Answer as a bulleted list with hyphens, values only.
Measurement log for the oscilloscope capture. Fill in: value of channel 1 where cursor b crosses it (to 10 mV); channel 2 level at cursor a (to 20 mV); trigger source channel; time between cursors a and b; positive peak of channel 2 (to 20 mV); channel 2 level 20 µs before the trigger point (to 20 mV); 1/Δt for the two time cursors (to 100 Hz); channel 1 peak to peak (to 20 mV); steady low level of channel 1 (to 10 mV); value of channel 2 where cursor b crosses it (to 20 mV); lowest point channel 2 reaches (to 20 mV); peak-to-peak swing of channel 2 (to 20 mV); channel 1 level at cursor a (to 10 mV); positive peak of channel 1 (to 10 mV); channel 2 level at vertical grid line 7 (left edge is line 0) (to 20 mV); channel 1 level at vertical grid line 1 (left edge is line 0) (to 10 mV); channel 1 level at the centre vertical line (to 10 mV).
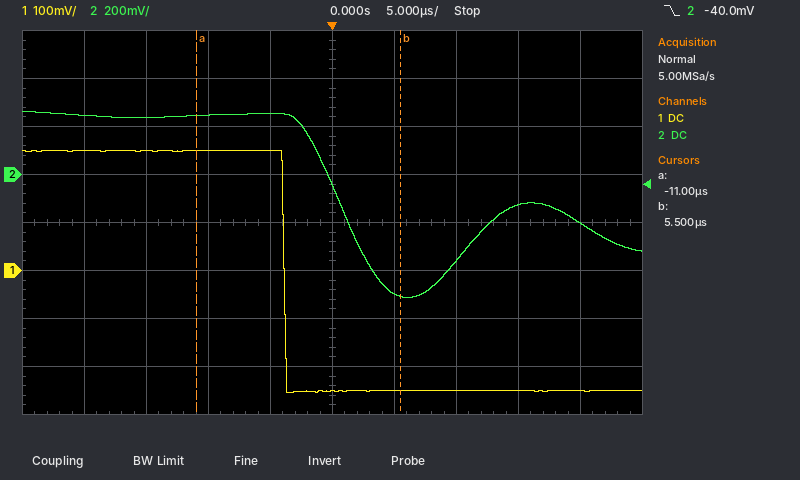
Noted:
- -250 mV
- 240 mV
- channel 2
- 16.5 µs
- 260 mV
- 240 mV
- 60.6 kHz
- 500 mV
- -250 mV
- -500 mV
- -520 mV
- 780 mV
- 250 mV
- 250 mV
- -360 mV
- 250 mV
- -250 mV
